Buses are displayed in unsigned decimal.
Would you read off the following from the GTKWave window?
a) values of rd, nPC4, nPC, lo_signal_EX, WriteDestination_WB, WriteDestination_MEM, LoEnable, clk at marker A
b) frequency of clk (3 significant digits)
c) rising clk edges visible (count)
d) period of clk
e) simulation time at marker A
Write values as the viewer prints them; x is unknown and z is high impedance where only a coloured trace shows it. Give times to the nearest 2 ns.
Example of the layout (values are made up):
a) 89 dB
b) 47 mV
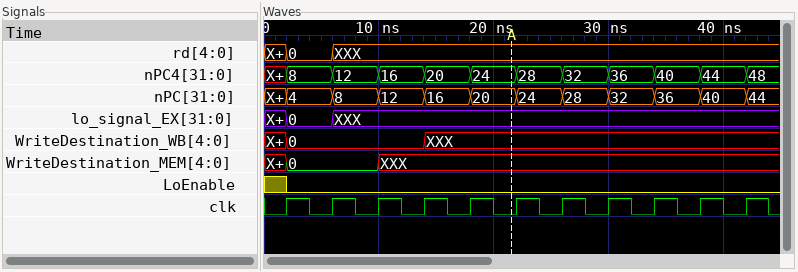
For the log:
a) rd=XXX, nPC4=24, nPC=20, lo_signal_EX=XXX, WriteDestination_WB=XXX, WriteDestination_MEM=XXX, LoEnable=0, clk=0
b) 250 MHz
c) 11
d) 4 ns
e) 22 ns
